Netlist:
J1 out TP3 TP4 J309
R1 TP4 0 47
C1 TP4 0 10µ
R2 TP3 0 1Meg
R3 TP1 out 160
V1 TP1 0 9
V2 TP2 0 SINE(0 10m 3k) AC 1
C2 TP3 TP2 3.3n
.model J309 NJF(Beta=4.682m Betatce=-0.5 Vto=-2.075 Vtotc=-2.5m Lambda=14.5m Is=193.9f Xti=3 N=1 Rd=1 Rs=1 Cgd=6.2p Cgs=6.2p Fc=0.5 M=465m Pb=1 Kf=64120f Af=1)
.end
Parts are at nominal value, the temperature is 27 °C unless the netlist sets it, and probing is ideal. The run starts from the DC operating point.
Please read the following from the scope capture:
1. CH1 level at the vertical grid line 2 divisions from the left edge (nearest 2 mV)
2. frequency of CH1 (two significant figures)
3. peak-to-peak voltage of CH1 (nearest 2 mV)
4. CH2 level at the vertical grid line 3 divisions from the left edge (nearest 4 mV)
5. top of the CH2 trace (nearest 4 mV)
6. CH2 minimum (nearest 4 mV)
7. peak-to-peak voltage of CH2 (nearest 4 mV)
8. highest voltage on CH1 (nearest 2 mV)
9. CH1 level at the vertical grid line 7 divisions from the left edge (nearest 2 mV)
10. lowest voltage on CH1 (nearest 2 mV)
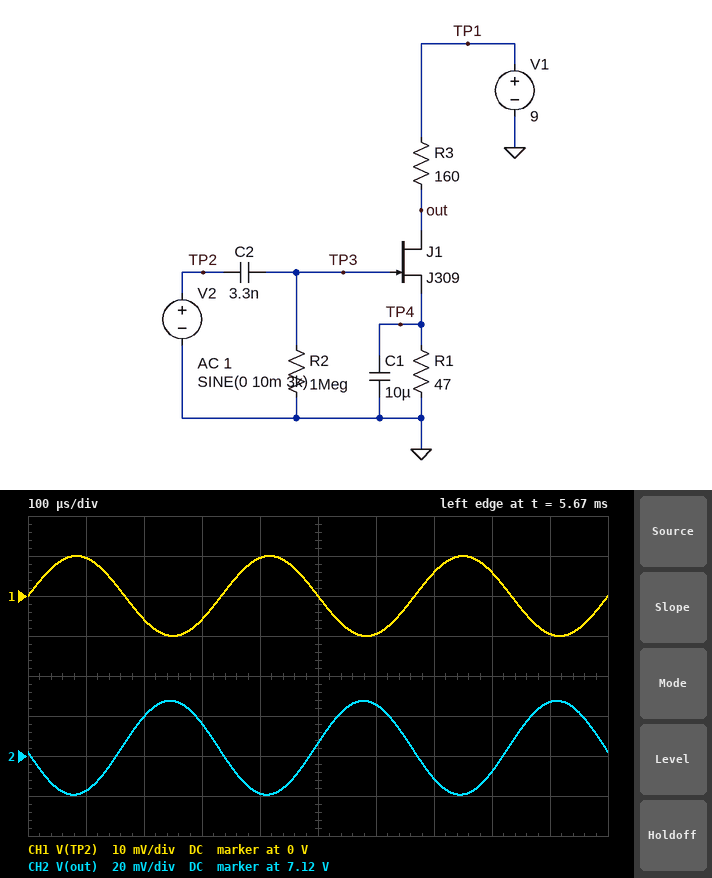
-6 mV
3.0 kHz
20 mV
7.136 V
7.148 V
7.100 V
48 mV
10 mV
6 mV
-10 mV
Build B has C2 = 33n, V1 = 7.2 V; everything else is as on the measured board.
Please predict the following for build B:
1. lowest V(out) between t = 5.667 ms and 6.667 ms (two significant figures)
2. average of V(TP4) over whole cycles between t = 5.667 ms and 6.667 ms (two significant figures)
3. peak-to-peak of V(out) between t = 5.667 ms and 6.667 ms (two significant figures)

5.3 V
540 mV
46 mV
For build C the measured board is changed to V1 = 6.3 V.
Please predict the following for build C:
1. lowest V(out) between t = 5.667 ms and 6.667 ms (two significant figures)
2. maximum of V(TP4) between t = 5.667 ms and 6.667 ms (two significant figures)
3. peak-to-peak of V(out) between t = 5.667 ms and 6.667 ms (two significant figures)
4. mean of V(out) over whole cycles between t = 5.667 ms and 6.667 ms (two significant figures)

4.4 V
540 mV
46 mV
4.5 V
